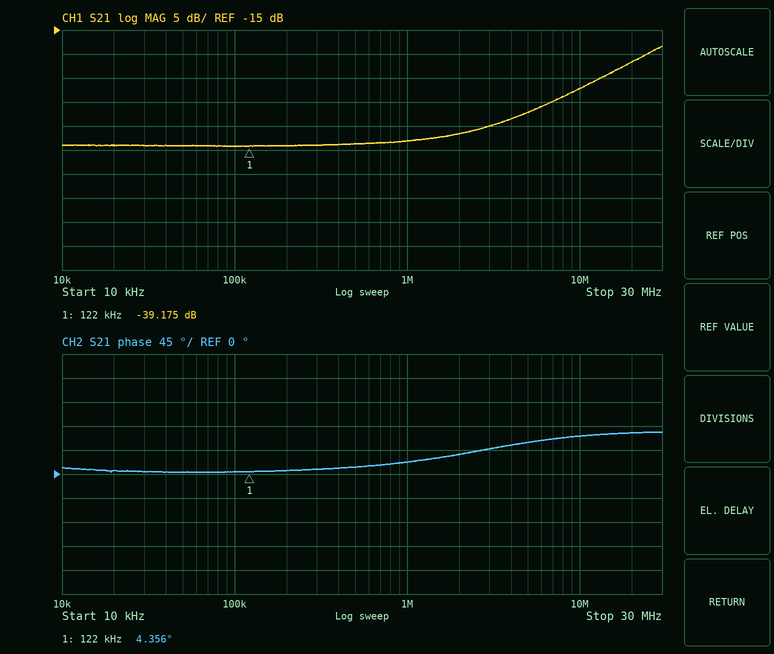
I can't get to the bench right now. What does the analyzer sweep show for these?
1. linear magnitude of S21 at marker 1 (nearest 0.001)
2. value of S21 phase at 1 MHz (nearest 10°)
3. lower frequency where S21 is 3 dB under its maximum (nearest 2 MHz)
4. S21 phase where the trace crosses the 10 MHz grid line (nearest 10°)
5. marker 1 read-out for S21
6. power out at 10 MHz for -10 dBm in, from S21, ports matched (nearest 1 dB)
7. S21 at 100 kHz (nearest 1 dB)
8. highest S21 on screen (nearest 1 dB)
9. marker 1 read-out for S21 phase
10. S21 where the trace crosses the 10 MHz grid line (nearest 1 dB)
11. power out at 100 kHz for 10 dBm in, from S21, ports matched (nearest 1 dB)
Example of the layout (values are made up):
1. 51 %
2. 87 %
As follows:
1. 0.011
2. 20°
3. 20 MHz
4. 70°
5. -39.175 dB
6. -37 dBm
7. -39 dB
8. -18 dB
9. 4.356°
10. -27 dB
11. -29 dBm
